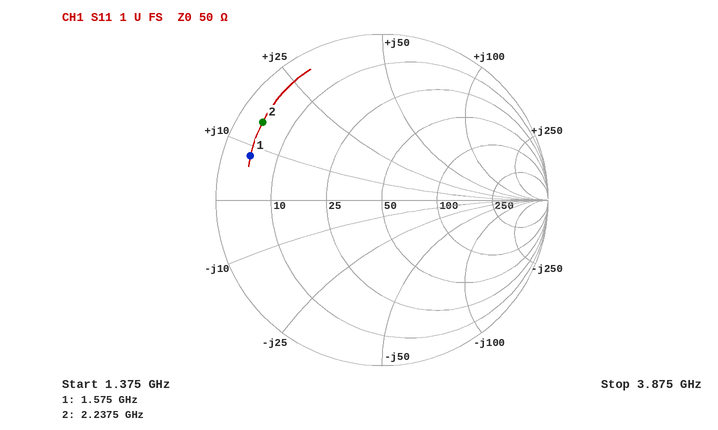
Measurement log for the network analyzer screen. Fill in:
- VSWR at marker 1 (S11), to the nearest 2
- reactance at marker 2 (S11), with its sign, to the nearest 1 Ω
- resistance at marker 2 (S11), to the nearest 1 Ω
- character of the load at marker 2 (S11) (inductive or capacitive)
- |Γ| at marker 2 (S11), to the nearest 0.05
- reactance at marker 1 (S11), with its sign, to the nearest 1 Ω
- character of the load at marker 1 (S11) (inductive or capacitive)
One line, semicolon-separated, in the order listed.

12; +15 Ω; 4 Ω; inductive; 0.85; +8 Ω; inductive
